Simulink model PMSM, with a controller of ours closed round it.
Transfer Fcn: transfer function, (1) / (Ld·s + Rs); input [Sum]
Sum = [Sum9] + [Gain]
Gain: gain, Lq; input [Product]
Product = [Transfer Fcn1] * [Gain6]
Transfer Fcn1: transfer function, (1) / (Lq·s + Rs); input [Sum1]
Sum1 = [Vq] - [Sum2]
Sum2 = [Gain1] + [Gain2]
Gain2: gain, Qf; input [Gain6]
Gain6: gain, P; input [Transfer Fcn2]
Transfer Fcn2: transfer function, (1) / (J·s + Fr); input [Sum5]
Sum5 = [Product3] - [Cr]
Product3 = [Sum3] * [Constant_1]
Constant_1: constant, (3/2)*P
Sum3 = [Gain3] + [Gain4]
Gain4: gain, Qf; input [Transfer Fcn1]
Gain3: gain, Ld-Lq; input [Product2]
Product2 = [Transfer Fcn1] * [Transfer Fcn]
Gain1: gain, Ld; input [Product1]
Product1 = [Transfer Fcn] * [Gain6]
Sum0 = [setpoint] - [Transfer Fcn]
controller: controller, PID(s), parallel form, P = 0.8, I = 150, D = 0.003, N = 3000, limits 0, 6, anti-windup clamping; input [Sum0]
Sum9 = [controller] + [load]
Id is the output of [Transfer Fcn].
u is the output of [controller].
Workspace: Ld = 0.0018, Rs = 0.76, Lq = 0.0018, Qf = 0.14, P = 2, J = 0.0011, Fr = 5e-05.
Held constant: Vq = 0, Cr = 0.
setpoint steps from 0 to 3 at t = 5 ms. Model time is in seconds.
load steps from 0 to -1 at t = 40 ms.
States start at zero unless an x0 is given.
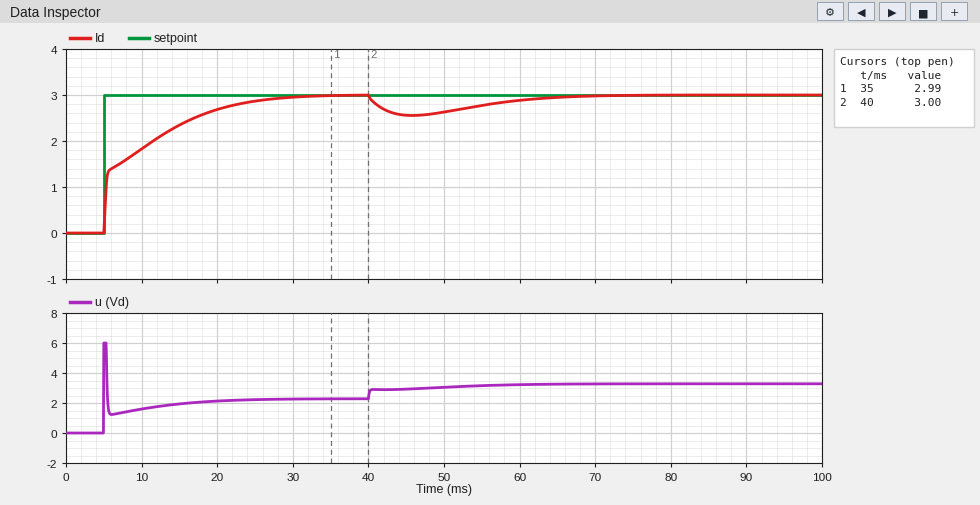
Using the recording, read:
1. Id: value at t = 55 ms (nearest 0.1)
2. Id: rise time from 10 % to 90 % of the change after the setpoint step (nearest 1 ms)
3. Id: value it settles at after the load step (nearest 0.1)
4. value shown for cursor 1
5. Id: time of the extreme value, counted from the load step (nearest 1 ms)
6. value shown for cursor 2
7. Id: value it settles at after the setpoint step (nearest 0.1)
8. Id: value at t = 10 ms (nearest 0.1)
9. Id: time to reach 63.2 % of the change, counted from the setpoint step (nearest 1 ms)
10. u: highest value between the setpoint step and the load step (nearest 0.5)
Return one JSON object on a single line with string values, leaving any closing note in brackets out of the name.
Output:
{"Id: value at t = 55 ms": "2.8", "Id: rise time from 10 % to 90 % of the change after the setpoint step": "15 ms", "Id: value it settles at after the load step": "3.0", "value shown for cursor 1": "2.99", "Id: time of the extreme value, counted from the load step": "6 ms", "value shown for cursor 2": "3.00", "Id: value it settles at after the setpoint step": "3.0", "Id: value at t = 10 ms": "1.8", "Id: time to reach 63.2 % of the change, counted from the setpoint step": "6 ms", "u: highest value between the setpoint step and the load step": "6.0"}
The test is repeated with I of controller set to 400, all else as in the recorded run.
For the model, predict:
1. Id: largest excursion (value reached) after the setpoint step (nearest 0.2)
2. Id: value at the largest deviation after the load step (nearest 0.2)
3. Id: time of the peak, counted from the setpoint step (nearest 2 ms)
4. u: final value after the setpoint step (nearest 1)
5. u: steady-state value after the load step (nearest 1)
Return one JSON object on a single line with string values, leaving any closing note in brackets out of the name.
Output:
{"Id: largest excursion (value reached) after the setpoint step": "3.2", "Id: value at the largest deviation after the load step": "2.6", "Id: time of the peak, counted from the setpoint step": "14 ms", "u: final value after the setpoint step": "2", "u: steady-state value after the load step": "3"}
